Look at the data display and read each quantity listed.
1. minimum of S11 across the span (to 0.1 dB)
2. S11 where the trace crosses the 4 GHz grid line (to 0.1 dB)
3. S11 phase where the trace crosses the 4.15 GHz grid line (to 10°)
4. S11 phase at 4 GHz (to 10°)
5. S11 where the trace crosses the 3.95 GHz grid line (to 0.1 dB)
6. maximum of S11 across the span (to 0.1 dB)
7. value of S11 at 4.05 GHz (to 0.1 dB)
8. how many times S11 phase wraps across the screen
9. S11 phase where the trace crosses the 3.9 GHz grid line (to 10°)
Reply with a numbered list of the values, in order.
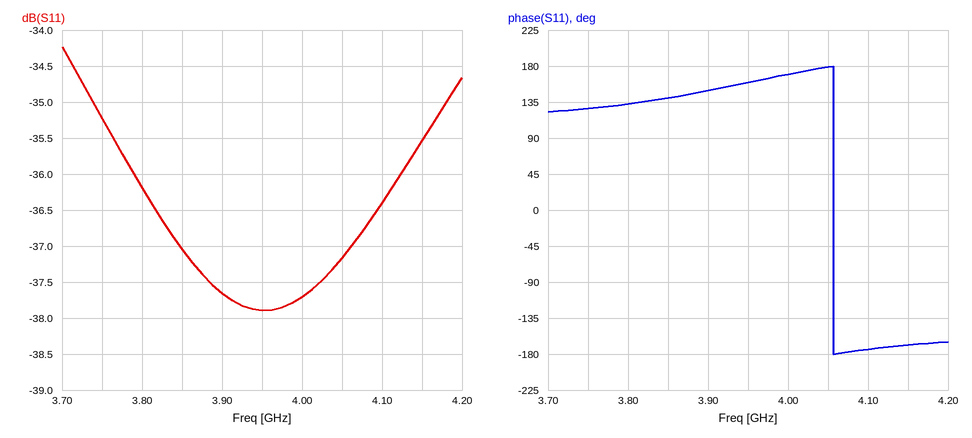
1. -37.9 dB
2. -37.7 dB
3. -170°
4. 170°
5. -37.9 dB
6. -34.2 dB
7. -37.2 dB
8. 1
9. 150°
